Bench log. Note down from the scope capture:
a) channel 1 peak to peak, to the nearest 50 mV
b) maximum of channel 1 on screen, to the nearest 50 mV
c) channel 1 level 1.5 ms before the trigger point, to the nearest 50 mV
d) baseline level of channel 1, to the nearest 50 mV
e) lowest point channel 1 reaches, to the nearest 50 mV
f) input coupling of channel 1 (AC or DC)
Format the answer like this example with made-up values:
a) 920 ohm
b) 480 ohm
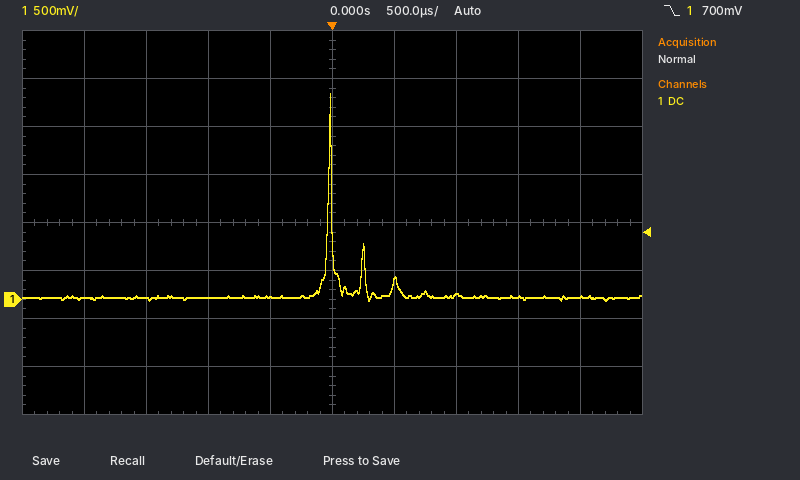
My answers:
a) 2.15 V
b) 2.15 V
c) 0 mV
d) 0 mV
e) 0 mV
f) DC
